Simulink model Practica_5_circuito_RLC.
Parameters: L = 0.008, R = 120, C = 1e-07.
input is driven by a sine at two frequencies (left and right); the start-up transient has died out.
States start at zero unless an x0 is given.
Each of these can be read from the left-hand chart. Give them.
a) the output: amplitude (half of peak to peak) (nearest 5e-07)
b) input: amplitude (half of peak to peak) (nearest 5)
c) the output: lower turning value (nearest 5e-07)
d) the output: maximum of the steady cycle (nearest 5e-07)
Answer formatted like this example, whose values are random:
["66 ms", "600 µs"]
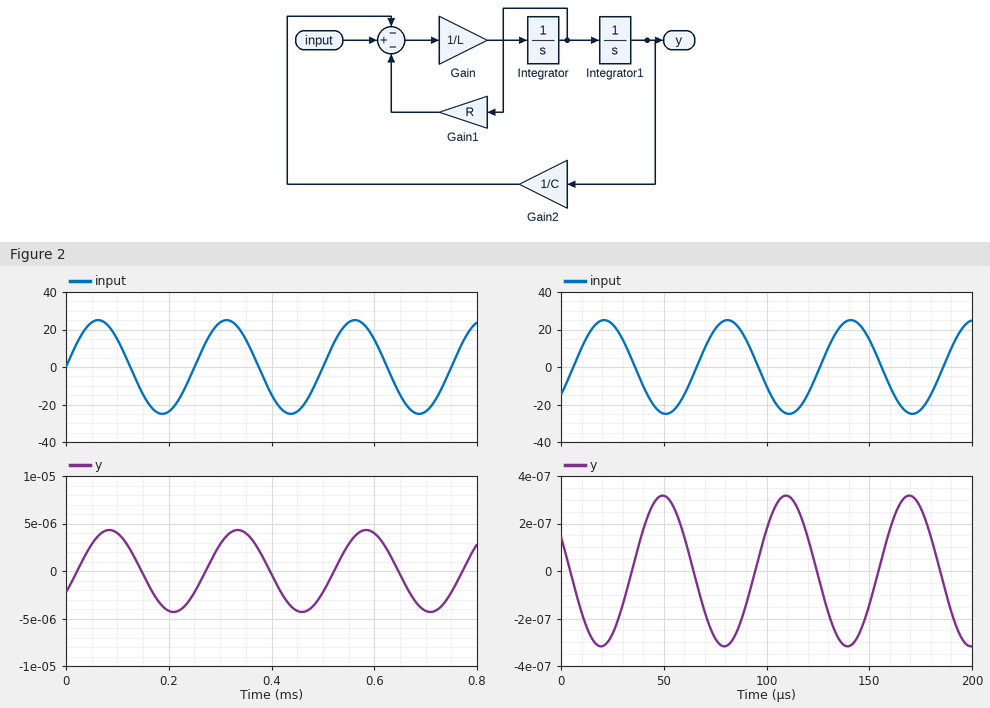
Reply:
["0.0000045", "25", "-0.0000045", "0.0000045"]
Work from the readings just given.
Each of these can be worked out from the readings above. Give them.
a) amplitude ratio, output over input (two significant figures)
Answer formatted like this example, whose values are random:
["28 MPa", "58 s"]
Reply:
["0.00000018"]
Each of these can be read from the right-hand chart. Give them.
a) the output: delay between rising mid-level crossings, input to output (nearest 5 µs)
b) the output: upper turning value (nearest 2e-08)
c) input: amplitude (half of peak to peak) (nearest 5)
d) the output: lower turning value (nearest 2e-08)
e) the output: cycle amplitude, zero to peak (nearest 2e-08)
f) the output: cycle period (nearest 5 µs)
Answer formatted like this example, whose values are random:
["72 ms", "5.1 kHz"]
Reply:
["30 µs", "0.00000032", "25", "-0.00000032", "0.00000032", "60 µs"]
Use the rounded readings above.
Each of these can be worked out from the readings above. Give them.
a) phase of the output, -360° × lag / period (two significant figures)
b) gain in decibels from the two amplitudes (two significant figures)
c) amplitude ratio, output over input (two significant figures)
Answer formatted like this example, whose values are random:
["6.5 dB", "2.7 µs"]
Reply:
["-180°", "-160 dB", "0.000000013"]
